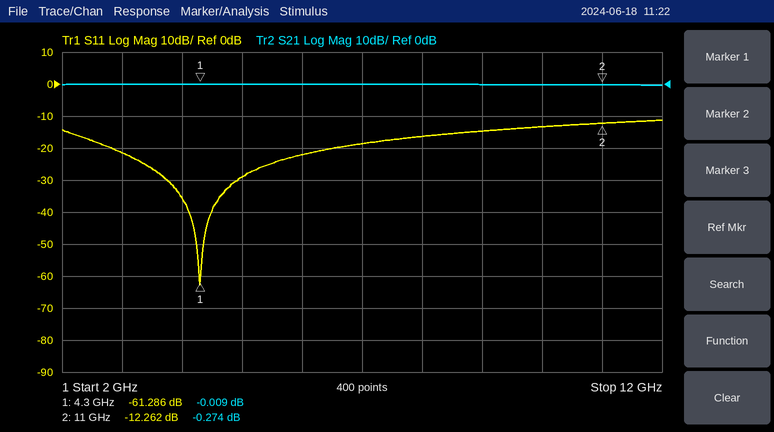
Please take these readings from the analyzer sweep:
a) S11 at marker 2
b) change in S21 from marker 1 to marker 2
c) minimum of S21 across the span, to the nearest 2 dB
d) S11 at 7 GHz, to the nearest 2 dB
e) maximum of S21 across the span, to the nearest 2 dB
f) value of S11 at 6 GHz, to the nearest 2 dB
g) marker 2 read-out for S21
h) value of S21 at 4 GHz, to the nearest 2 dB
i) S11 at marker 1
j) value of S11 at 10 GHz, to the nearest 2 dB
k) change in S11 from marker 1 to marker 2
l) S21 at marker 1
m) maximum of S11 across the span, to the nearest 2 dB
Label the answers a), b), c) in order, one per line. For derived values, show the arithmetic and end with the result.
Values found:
a) -12.262 dB
b) -0.274 − (-0.009) = -0.265 dB
c) 0 dB
d) -18 dB
e) 0 dB
f) -22 dB
g) -0.274 dB
h) 0 dB
i) -61.286 dB
j) -14 dB
k) -12.262 − (-61.286) = 49.024 dB
l) -0.009 dB
m) -12 dB
